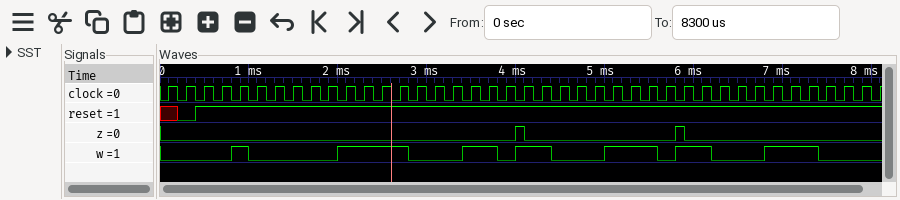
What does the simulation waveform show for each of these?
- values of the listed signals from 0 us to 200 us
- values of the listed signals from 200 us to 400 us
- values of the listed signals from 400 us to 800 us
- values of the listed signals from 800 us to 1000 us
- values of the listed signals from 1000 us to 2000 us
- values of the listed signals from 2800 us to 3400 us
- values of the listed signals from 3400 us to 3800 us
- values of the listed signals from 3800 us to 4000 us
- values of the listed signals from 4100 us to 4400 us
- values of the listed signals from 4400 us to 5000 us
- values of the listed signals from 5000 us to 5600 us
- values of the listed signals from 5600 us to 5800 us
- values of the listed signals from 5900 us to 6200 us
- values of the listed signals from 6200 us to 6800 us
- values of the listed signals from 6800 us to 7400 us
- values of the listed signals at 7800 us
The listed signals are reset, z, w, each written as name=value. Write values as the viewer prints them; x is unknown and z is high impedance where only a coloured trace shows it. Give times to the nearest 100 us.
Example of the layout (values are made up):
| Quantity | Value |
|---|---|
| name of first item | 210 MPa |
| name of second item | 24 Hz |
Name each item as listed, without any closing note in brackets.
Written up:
| Quantity | Value |
|---|---|
| values of the listed signals from 0 us to 200 us | reset=x, z=0, w=0 |
| values of the listed signals from 200 us to 400 us | reset=0, z=0, w=0 |
| values of the listed signals from 400 us to 800 us | reset=1, z=0, w=0 |
| values of the listed signals from 800 us to 1000 us | reset=1, z=0, w=1 |
| values of the listed signals from 1000 us to 2000 us | reset=1, z=0, w=0 |
| values of the listed signals from 2800 us to 3400 us | reset=1, z=0, w=0 |
| values of the listed signals from 3400 us to 3800 us | reset=1, z=0, w=1 |
| values of the listed signals from 3800 us to 4000 us | reset=1, z=0, w=0 |
| values of the listed signals from 4100 us to 4400 us | reset=1, z=0, w=1 |
| values of the listed signals from 4400 us to 5000 us | reset=1, z=0, w=0 |
| values of the listed signals from 5000 us to 5600 us | reset=1, z=0, w=1 |
| values of the listed signals from 5600 us to 5800 us | reset=1, z=0, w=0 |
| values of the listed signals from 5900 us to 6200 us | reset=1, z=0, w=1 |
| values of the listed signals from 6200 us to 6800 us | reset=1, z=0, w=0 |
| values of the listed signals from 6800 us to 7400 us | reset=1, z=0, w=1 |
| values of the listed signals at 7800 us | reset=1, z=0, w=0 |
